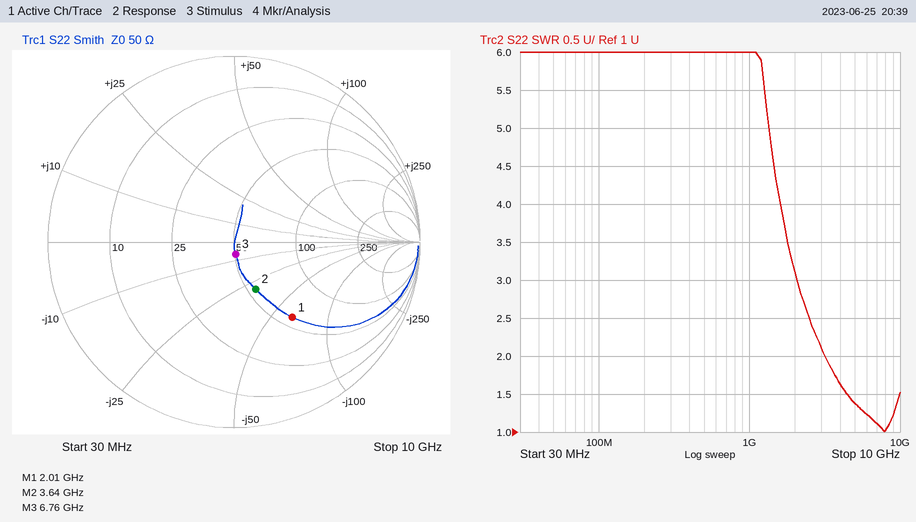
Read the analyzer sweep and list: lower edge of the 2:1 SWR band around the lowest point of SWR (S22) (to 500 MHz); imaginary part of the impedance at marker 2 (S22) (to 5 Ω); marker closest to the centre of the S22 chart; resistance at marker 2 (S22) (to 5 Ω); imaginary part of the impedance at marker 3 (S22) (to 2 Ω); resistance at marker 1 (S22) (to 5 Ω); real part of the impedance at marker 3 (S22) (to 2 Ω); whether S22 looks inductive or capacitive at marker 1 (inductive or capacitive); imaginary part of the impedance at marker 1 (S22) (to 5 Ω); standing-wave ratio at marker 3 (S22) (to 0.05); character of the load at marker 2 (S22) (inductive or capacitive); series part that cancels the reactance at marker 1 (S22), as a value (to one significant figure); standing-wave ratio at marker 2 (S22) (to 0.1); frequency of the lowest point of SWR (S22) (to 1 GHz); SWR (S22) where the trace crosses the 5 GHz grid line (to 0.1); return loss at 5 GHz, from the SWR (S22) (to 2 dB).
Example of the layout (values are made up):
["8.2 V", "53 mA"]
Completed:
["3.0 GHz", "-30 Ω", "marker 3", "55 Ω", "-6 Ω", "60 Ω", "50 Ω", "capacitive", "-65 Ω", "1.15", "capacitive", "5 nH", "1.8", "8 GHz", "1.4", "16 dB"]
